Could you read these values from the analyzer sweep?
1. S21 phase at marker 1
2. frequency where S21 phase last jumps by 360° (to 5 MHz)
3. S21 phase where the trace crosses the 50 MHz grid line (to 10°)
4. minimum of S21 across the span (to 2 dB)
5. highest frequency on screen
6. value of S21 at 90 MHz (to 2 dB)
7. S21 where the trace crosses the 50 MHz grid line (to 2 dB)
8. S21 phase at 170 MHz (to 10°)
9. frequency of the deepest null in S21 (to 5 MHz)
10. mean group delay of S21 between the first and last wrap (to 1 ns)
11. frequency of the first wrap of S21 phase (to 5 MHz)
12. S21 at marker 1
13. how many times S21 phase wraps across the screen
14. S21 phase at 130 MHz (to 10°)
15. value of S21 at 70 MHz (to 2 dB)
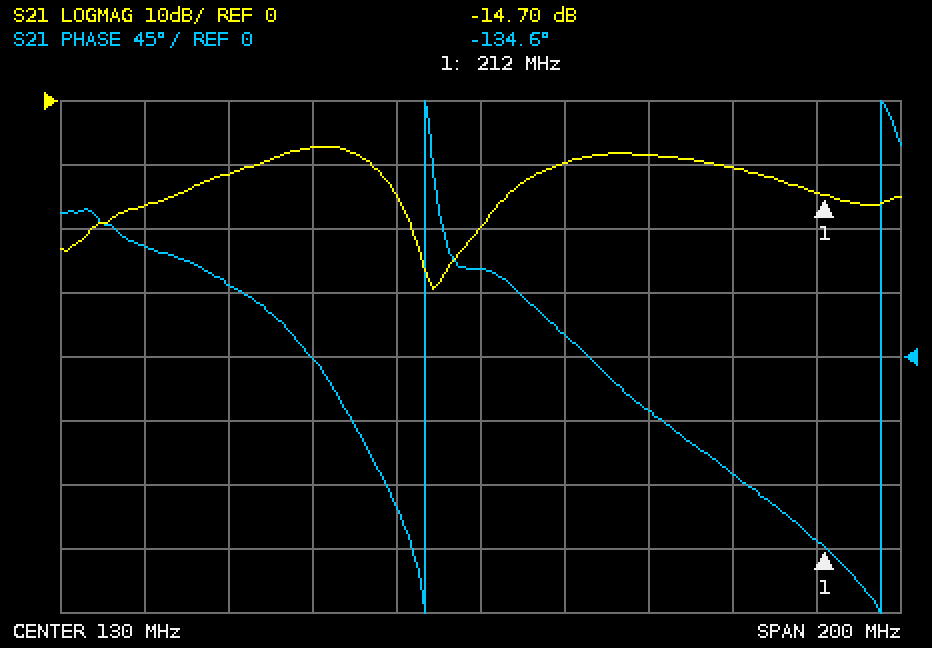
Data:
-134.6°
225 MHz
80°
-30 dB
230 MHz
-8 dB
-16 dB
-40°
120 MHz
9 ns
115 MHz
-14.70 dB
2
60°
-12 dB
